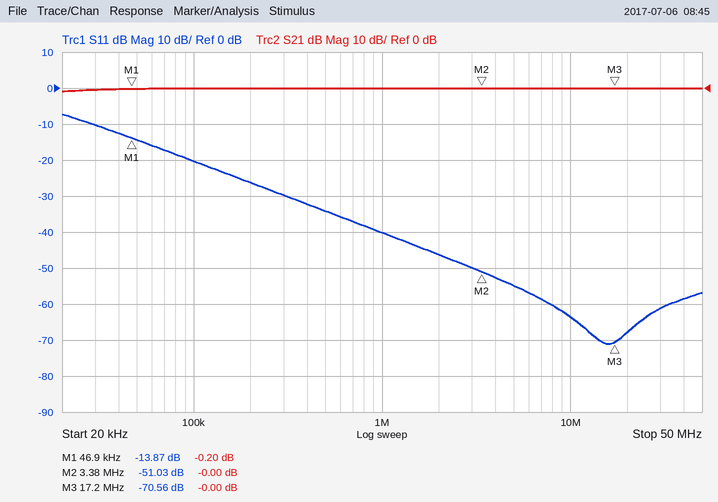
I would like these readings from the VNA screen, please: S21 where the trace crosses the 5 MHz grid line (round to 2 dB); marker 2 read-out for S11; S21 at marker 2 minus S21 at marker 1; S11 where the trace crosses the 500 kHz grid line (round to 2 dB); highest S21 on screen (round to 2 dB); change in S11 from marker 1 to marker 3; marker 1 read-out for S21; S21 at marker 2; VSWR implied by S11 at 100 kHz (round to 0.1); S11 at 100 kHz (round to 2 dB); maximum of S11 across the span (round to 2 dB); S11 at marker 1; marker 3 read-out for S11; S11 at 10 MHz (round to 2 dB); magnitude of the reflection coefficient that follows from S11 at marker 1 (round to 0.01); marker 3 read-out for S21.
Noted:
0 dB
-51.03 dB
0.20 dB
-34 dB
0 dB
-56.69 dB
-0.20 dB
-0.00 dB
1.2
-20 dB
-8 dB
-13.87 dB
-70.56 dB
-64 dB
0.20
-0.00 dB
